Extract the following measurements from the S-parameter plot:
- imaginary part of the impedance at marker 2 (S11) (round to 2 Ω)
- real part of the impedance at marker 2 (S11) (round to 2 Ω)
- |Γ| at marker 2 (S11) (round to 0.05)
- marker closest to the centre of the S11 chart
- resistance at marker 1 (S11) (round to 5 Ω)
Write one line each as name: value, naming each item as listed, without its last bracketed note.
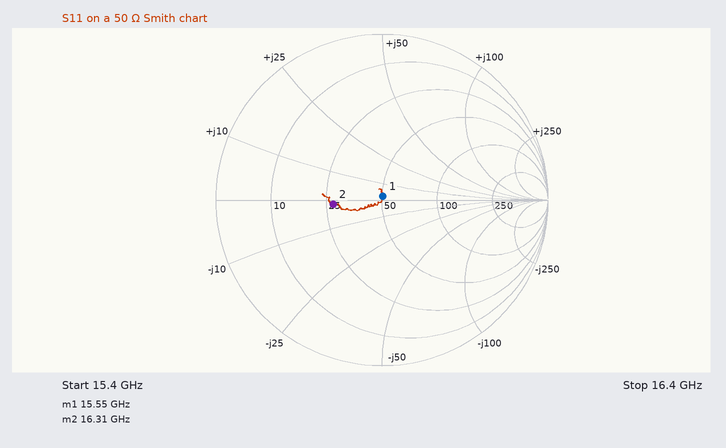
imaginary part of the impedance at marker 2 (S11): -2 Ω
real part of the impedance at marker 2 (S11): 28 Ω
|Γ| at marker 2 (S11): 0.30
marker closest to the centre of the S11 chart: marker 1
resistance at marker 1 (S11): 50 Ω
